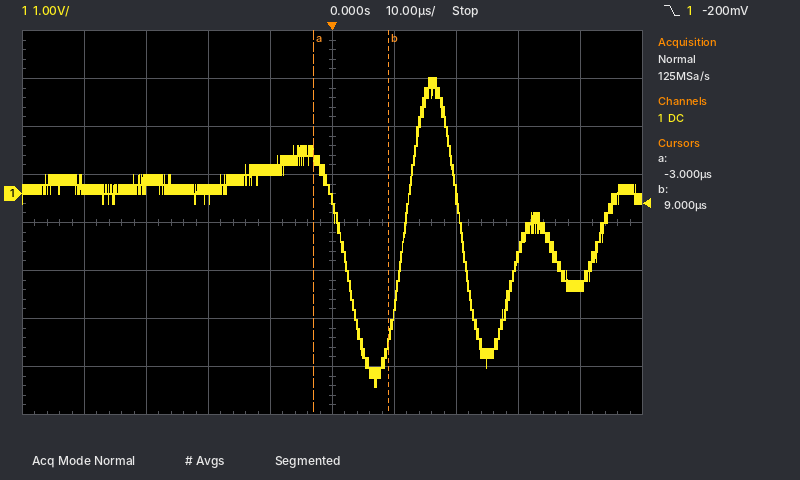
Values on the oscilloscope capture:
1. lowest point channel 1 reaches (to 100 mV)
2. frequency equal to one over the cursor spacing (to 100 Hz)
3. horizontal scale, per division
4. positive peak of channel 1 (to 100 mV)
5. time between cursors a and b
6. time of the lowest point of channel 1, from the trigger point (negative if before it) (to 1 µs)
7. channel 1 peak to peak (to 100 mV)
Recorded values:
-4.0 V
83.3 kHz
10 µs
2.4 V
12 µs
+7 µs
6.4 V
